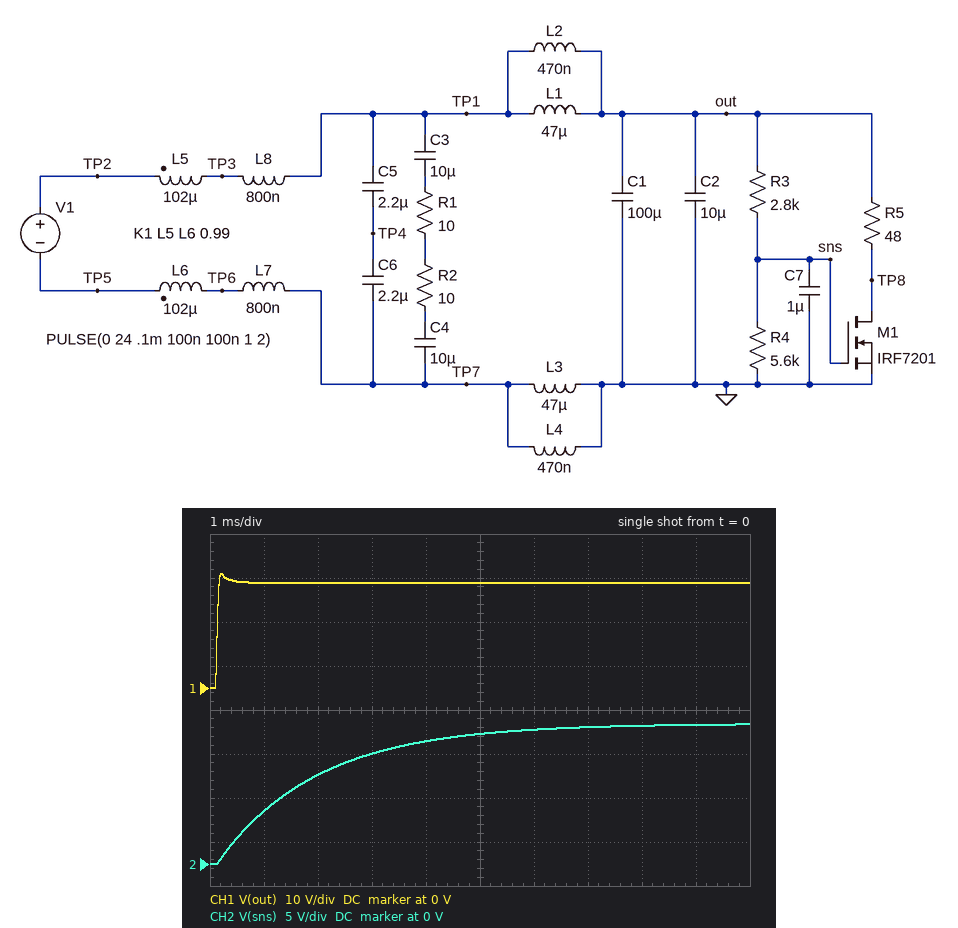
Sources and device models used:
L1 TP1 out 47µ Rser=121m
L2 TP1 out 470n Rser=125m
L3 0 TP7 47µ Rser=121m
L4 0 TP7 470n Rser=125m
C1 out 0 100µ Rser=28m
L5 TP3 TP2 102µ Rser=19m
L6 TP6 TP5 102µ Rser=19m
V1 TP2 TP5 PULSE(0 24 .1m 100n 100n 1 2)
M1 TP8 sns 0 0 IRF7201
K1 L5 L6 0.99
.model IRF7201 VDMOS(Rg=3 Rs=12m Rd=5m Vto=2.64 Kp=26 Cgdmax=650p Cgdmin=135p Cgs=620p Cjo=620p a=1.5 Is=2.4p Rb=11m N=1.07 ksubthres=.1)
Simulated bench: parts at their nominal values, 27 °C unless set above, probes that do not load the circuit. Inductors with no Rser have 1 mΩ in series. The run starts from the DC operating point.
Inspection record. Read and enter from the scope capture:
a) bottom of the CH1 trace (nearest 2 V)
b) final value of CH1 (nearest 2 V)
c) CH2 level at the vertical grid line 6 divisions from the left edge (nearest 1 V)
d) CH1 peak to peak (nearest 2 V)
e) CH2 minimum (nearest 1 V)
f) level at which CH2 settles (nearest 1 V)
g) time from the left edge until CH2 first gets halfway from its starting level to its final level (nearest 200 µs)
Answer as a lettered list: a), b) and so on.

a) 0 V
b) 24 V
c) 15 V
d) 26 V
e) 0 V
f) 16 V
g) 1.4 ms
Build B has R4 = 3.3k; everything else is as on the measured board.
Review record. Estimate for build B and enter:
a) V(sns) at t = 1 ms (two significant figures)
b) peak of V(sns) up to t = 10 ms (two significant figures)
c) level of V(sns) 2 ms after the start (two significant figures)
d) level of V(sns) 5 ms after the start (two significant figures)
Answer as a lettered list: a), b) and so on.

a) 5.7 V
b) 13 V
c) 9.2 V
d) 12 V
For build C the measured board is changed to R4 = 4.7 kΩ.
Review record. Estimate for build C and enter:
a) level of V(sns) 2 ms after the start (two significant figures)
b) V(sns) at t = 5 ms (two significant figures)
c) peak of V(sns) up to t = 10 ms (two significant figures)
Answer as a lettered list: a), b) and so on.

a) 9.9 V
b) 14 V
c) 15 V
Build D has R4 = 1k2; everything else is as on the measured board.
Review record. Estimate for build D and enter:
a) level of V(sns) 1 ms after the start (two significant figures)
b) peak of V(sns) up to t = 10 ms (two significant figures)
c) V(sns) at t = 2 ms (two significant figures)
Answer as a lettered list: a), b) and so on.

a) 4.7 V
b) 7.2 V
c) 6.4 V
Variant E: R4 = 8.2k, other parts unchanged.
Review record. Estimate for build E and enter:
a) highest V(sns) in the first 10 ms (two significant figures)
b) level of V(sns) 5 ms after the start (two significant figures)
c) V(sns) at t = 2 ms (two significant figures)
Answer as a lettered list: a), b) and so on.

a) 18 V
b) 16 V
c) 11 V
